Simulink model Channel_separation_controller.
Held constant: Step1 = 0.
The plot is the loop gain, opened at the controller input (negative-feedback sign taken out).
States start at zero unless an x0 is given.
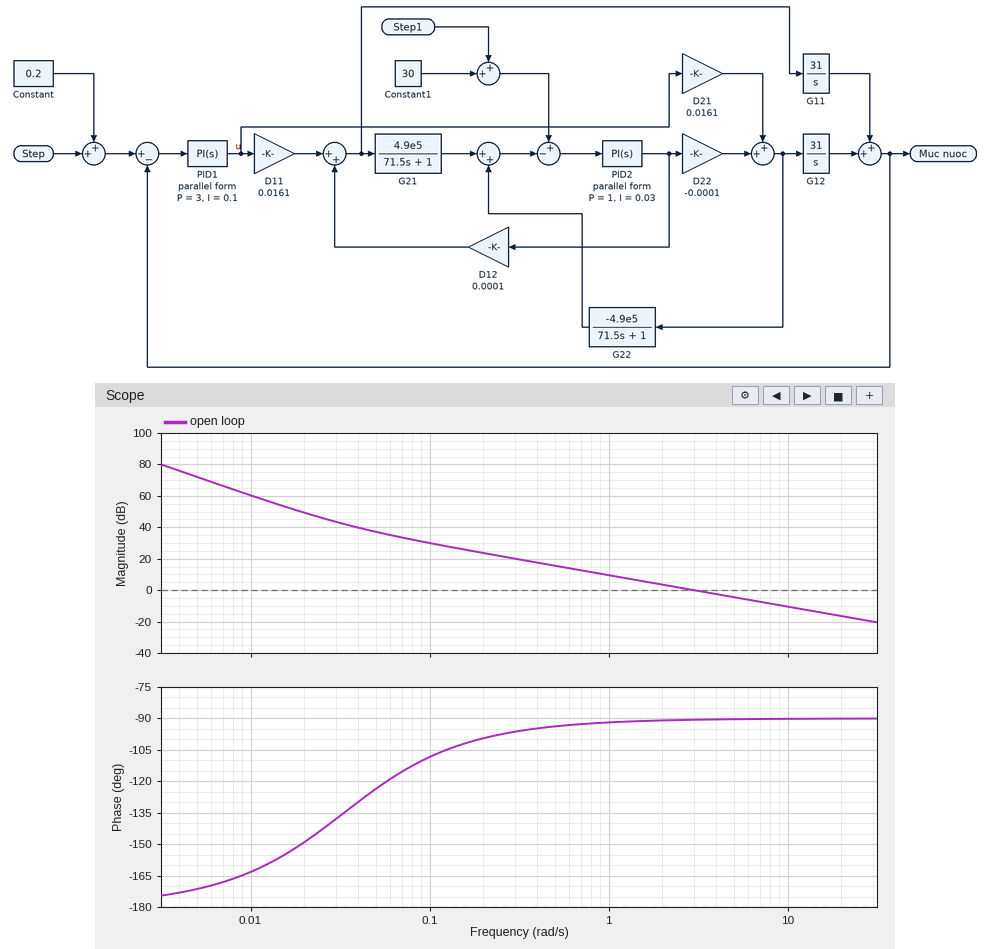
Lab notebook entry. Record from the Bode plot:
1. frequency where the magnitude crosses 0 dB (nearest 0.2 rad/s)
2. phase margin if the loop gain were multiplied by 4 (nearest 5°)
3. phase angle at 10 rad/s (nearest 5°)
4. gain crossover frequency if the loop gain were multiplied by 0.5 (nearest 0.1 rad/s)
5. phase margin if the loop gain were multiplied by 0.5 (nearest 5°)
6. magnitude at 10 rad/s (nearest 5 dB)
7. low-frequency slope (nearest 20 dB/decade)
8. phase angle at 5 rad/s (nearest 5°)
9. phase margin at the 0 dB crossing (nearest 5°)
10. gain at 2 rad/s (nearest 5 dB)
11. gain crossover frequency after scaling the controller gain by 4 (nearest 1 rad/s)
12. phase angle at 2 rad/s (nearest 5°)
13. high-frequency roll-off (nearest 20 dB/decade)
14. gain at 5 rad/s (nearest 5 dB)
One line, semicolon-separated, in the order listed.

3.0 rad/s; 90°; -90°; 1.5 rad/s; 90°; -10 dB; -40 dB/decade; -90°; 90°; 5 dB; 12 rad/s; -90°; -20 dB/decade; -5 dB
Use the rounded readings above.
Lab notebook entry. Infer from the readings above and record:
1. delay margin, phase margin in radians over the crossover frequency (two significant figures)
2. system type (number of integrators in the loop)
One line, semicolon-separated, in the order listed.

0.52 s; 2
